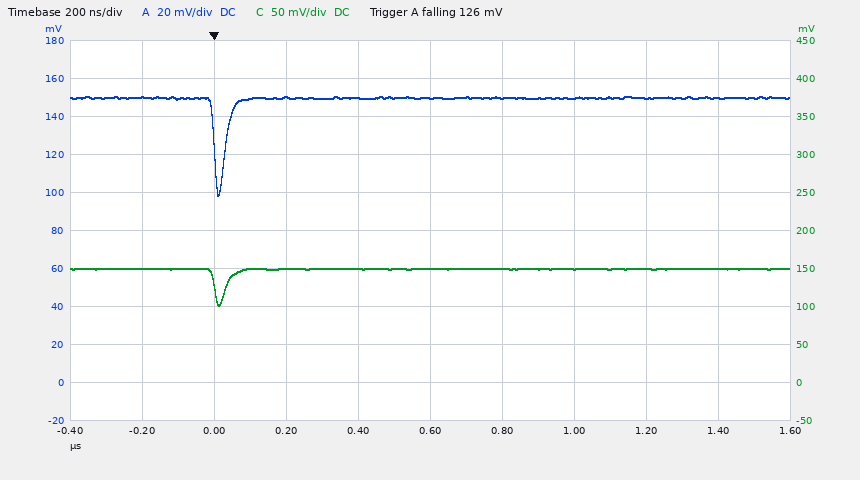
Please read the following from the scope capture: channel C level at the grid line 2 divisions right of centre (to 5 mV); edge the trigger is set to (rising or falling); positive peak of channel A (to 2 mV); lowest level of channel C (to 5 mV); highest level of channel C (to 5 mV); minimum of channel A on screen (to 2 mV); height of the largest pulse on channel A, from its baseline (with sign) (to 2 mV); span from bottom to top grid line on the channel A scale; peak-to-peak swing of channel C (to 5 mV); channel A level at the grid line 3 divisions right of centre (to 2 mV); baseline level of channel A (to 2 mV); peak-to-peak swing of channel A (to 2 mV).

150 mV
falling
150 mV
100 mV
150 mV
98 mV
-52 mV
200 mV
50 mV
150 mV
150 mV
52 mV
